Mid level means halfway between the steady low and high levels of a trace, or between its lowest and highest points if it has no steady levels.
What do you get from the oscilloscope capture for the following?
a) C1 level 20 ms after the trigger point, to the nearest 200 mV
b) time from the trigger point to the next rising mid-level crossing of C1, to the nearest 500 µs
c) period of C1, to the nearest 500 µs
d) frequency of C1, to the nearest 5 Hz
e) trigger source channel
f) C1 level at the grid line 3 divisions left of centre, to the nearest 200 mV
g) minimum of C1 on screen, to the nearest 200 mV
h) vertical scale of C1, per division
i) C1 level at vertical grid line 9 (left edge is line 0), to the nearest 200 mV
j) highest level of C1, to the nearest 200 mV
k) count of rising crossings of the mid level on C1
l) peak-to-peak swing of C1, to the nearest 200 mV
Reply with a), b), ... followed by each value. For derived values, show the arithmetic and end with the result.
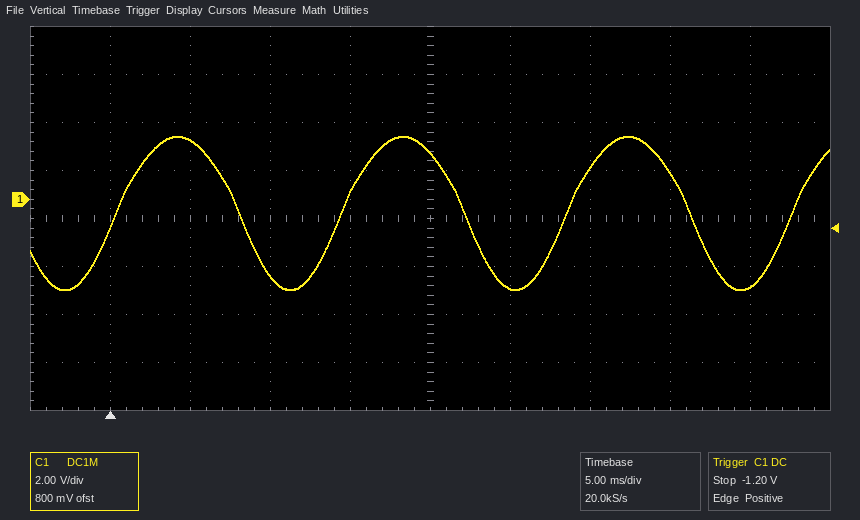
a) 2.0 V
b) 500 µs
c) 14.0 ms
d) 1 / 14.0 ms ≈ 71.4 Hz, so 70 Hz to the nearest 5 Hz
e) C1
f) 2.4 V
g) -3.8 V
h) 2 V
i) -3.6 V
j) 2.6 V
k) 4
l) 2.6 V − (-3.8 V) = 6.4 V
